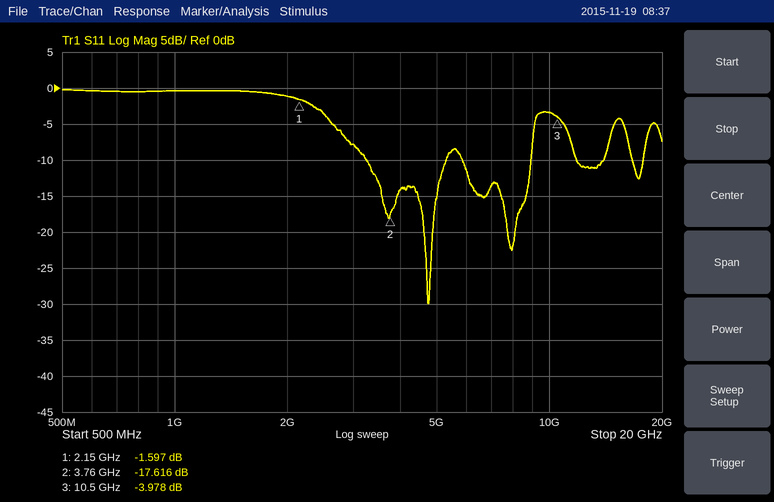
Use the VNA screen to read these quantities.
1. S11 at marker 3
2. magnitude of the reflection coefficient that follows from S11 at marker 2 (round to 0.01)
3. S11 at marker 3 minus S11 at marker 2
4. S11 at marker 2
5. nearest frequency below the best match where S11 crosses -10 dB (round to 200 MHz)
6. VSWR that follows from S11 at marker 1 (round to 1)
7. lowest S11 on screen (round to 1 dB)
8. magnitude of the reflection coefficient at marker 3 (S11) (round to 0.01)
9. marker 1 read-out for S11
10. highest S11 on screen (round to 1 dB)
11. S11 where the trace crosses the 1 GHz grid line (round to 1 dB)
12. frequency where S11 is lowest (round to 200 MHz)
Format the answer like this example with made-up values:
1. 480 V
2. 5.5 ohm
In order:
1. -3.978 dB
2. 0.13
3. 13.638 dB
4. -17.616 dB
5. 3.2 GHz
6. 11
7. -30 dB
8. 0.63
9. -1.597 dB
10. 0 dB
11. 0 dB
12. 4.8 GHz
